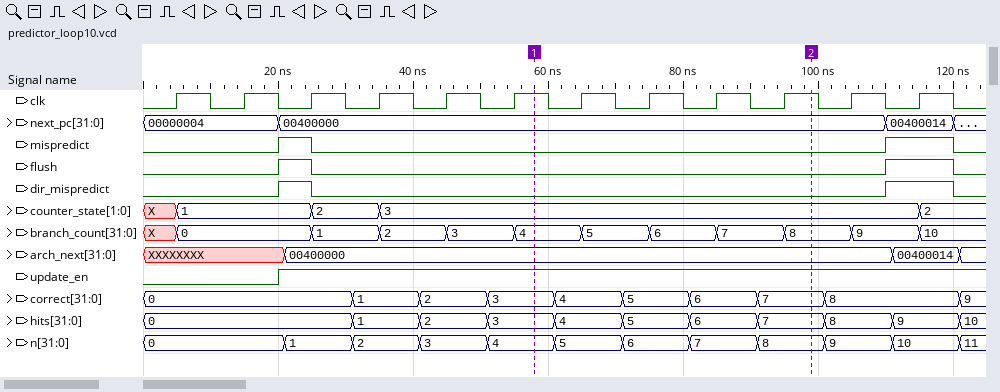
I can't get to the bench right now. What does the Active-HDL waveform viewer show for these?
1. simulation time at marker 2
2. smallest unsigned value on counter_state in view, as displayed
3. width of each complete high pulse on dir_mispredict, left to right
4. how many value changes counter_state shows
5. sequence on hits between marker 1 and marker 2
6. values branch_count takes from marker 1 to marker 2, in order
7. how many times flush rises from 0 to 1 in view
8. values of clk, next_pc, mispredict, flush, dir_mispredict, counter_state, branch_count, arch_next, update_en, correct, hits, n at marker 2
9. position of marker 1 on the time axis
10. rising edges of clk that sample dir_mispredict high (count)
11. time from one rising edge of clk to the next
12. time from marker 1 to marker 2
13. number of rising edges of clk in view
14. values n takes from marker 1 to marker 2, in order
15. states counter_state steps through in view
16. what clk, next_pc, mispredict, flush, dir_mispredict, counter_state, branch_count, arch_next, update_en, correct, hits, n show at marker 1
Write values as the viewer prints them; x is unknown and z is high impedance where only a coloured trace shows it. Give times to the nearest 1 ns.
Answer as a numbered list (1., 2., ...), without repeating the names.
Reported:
1. 99 ns
2. 1
3. 5 ns, 10 ns
4. 4
5. 3, 4, 5, 6, 7
6. 4, 5, 6, 7, 8
7. 2
8. clk=1, next_pc=00400000, mispredict=0, flush=0, dir_mispredict=0, counter_state=3, branch_count=8, arch_next=00400000, update_en=1, correct=7, hits=7, n=8
9. 58 ns
10. 2
11. 10 ns
12. 41 ns
13. 12
14. 4, 5, 6, 7, 8
15. X, 1, 2, 3, 2
16. clk=1, next_pc=00400000, mispredict=0, flush=0, dir_mispredict=0, counter_state=3, branch_count=4, arch_next=00400000, update_en=1, correct=3, hits=3, n=4
